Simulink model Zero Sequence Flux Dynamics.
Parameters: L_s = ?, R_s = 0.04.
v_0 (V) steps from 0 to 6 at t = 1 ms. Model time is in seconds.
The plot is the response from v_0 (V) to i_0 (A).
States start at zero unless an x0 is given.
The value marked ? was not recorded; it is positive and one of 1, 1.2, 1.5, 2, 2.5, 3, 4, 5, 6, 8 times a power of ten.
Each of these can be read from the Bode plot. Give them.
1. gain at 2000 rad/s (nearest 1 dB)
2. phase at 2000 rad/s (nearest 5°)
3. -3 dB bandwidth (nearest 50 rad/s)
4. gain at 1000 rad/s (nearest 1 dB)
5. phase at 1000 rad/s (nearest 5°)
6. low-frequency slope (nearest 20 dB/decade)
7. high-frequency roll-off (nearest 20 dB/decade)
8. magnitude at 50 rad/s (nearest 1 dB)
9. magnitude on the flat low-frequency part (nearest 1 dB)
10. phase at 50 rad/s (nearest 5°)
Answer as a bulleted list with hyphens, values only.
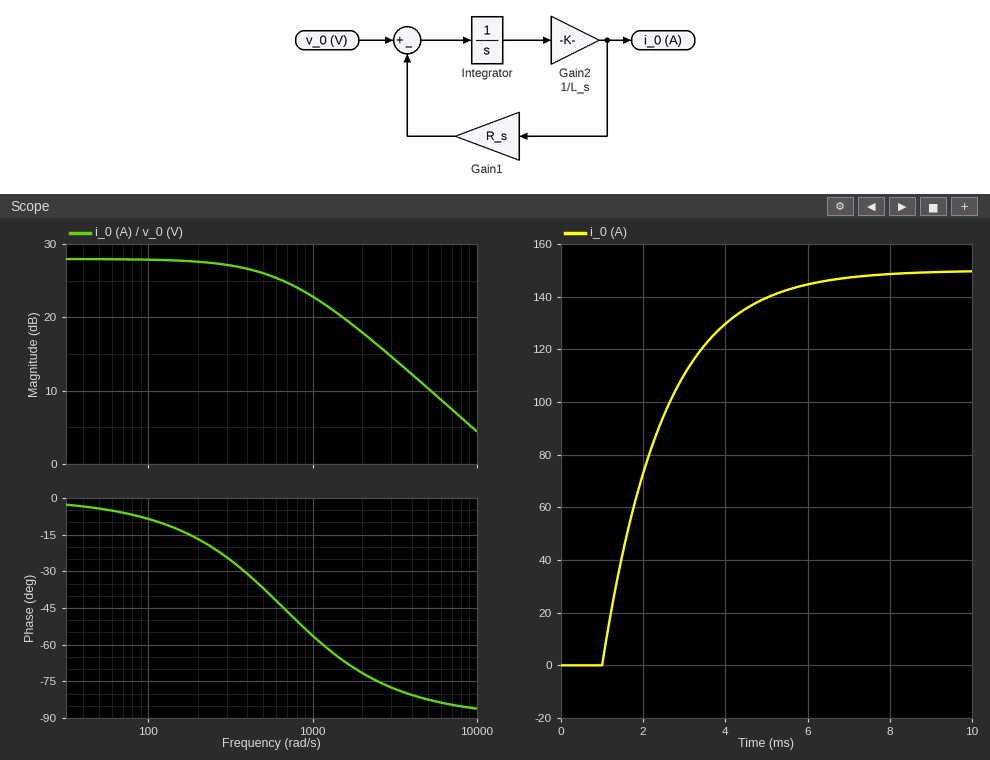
- 18 dB
- -70°
- 650 rad/s
- 23 dB
- -55°
- 0 dB/decade
- -20 dB/decade
- 28 dB
- 28 dB
- -5°
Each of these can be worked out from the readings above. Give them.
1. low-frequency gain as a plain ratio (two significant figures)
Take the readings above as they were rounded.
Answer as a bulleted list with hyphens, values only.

- 25
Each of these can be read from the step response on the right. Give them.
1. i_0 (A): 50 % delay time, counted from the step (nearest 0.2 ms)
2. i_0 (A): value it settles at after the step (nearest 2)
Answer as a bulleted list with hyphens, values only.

- 1.0 ms
- 150
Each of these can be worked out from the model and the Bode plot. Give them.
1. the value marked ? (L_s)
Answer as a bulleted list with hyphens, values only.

- 6e-05
